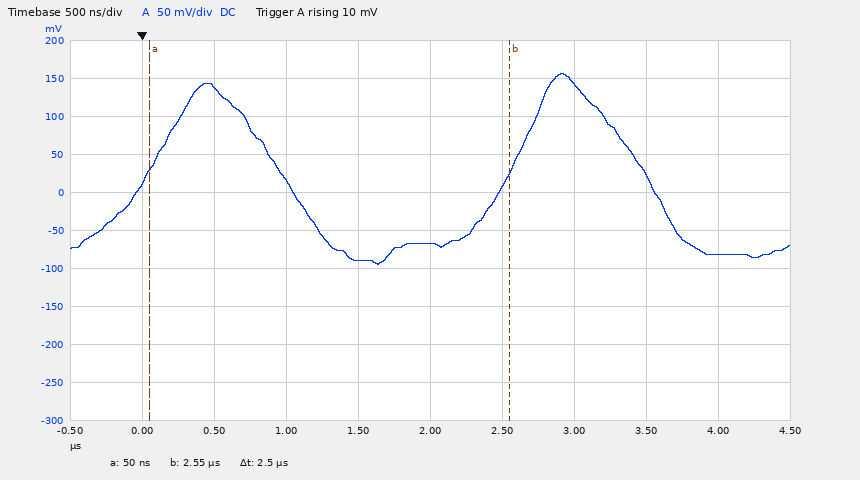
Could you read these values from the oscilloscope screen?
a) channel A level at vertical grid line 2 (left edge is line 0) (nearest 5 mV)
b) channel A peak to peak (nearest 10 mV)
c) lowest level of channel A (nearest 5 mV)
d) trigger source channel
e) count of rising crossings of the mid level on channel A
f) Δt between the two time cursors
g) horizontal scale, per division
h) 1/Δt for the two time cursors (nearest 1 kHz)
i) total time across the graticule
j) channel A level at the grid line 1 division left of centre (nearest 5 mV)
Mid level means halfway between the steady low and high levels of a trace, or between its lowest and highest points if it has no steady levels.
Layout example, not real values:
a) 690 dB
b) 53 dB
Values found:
a) 140 mV
b) 250 mV
c) -95 mV
d) channel A
e) 2
f) 2.5 µs
g) 500 ns
h) 400 kHz
i) 5 µs
j) -90 mV
